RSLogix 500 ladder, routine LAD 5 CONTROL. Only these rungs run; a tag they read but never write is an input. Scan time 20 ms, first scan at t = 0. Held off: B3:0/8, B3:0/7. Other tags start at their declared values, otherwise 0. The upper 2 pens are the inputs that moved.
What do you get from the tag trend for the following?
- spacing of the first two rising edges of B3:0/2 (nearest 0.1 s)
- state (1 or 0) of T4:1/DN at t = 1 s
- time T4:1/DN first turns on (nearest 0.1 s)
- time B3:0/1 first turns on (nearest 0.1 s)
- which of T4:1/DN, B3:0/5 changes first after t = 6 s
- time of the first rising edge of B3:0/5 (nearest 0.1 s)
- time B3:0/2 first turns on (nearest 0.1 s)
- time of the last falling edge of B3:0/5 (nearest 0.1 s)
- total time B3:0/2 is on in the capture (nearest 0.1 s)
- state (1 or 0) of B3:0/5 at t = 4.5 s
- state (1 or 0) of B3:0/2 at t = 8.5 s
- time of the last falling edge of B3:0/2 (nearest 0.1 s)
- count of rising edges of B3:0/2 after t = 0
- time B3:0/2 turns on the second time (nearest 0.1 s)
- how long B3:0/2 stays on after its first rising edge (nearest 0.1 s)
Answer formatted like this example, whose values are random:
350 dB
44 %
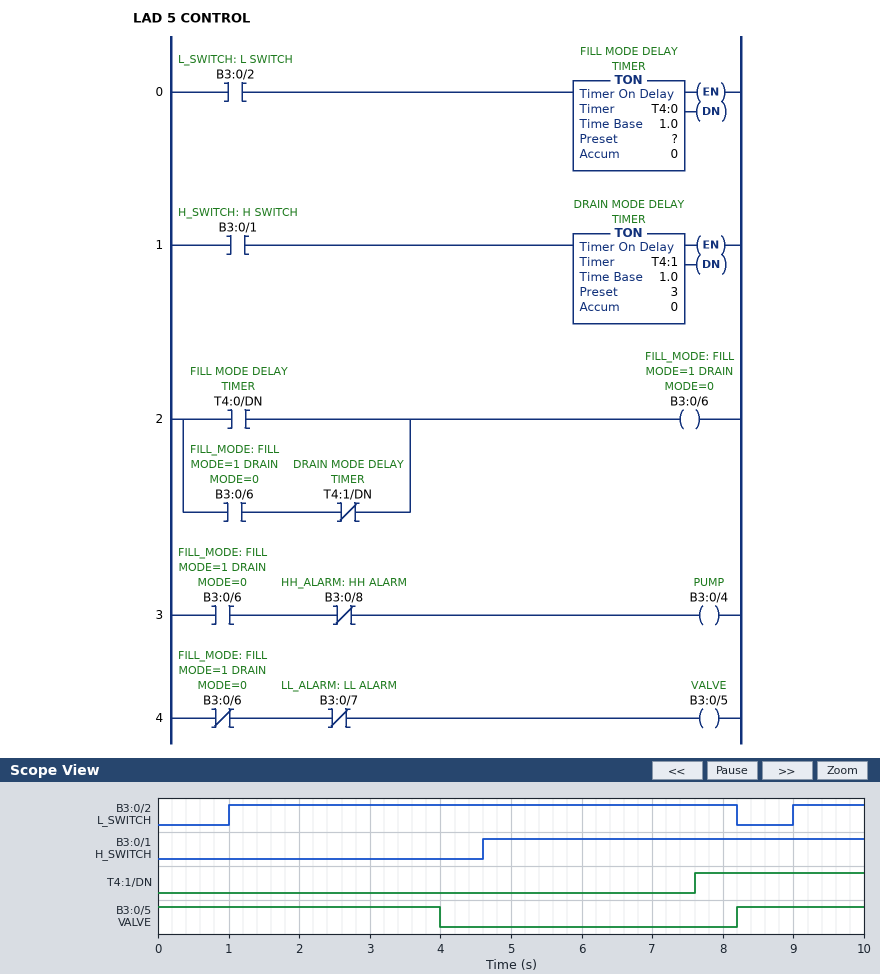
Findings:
8.0 s
0
7.6 s
4.6 s
T4:1/DN
8.2 s
1.0 s
4.0 s
8.2 s
0
0
8.2 s
2
9.0 s
7.2 s
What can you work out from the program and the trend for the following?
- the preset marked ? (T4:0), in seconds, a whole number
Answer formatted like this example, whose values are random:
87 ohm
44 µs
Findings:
3 s
